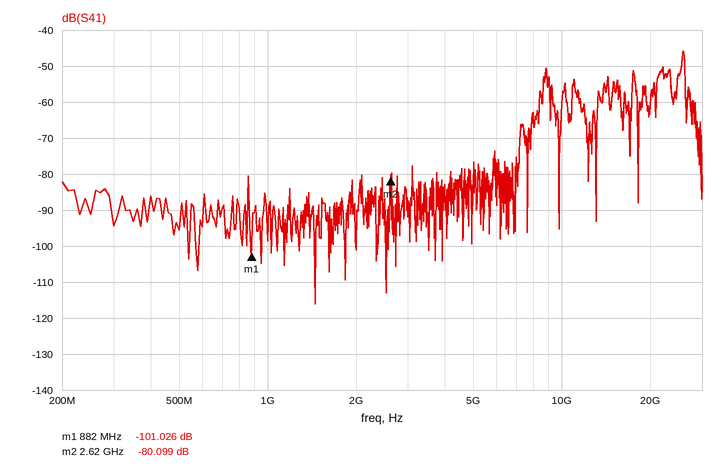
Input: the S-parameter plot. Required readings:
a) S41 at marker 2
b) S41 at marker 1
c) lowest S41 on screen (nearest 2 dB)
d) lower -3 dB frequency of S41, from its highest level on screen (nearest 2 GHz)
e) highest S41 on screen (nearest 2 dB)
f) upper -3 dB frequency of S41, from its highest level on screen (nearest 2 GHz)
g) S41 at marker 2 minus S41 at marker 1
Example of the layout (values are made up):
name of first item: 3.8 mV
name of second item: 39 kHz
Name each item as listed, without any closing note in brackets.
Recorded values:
S41 at marker 2: -80.099 dB
S41 at marker 1: -101.026 dB
lowest S41 on screen: -116 dB
lower -3 dB frequency of S41, from its highest level on screen: 26 GHz
highest S41 on screen: -46 dB
upper -3 dB frequency of S41, from its highest level on screen: 26 GHz
S41 at marker 2 minus S41 at marker 1: 20.927 dB
